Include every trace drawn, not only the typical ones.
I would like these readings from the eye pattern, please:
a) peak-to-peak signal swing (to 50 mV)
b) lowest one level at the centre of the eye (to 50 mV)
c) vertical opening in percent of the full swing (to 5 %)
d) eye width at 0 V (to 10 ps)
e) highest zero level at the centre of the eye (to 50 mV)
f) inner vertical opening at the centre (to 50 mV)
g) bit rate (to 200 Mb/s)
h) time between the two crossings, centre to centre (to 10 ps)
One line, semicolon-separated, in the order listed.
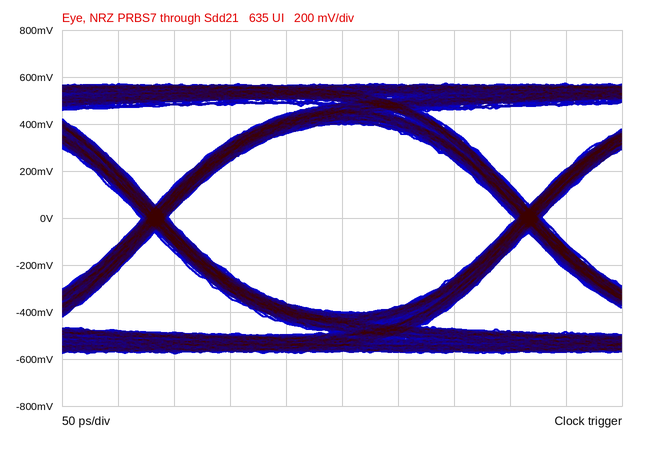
1.15 V; 400 mV; 70 %; 310 ps; -400 mV; 800 mV; 3.0 Gb/s; 330 ps
